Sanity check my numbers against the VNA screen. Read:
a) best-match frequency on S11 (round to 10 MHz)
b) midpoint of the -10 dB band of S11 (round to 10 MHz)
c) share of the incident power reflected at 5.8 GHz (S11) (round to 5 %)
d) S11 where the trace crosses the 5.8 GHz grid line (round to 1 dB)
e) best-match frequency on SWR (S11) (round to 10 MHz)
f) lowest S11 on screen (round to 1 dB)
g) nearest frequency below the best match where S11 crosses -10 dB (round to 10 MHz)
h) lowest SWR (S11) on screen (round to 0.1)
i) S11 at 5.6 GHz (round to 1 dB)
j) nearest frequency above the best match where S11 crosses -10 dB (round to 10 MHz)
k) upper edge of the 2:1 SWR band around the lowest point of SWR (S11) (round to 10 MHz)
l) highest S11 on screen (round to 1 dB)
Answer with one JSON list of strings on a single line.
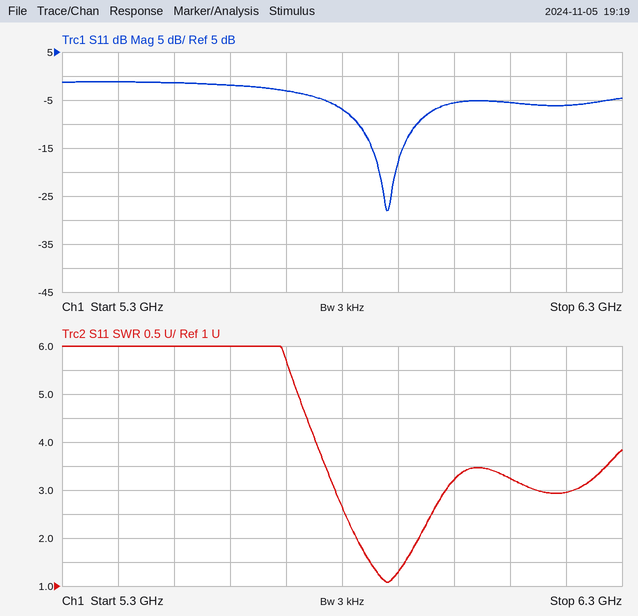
["5.88 GHz", "5.88 GHz", "20 %", "-7 dB", "5.88 GHz", "-28 dB", "5.83 GHz", "1.1", "-2 dB", "5.93 GHz", "5.94 GHz", "-1 dB"]
